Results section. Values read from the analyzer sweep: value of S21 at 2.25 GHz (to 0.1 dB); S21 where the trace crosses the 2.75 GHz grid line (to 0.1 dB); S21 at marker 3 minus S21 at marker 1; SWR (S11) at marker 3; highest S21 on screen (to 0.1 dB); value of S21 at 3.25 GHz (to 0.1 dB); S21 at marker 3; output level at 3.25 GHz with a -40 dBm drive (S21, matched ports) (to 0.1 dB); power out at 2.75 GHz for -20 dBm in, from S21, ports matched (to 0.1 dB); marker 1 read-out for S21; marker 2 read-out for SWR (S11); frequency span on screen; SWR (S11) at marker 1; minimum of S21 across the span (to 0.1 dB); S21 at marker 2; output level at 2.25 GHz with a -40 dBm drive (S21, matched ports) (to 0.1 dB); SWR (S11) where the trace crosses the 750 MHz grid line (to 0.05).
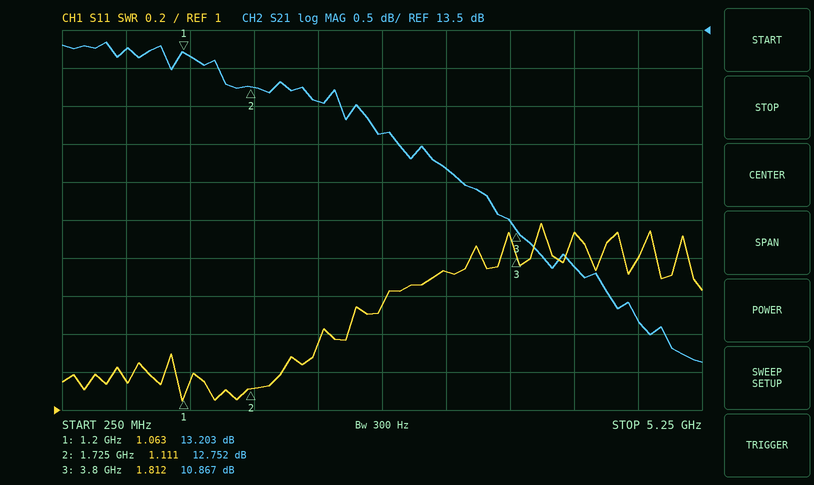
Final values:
12.6 dB
12.1 dB
-2.336 dB
1.812
13.3 dB
11.7 dB
10.867 dB
-28.3 dBm
-7.9 dBm
13.203 dB
1.111
5 GHz
1.063
9.1 dB
12.752 dB
-27.4 dBm
1.15
